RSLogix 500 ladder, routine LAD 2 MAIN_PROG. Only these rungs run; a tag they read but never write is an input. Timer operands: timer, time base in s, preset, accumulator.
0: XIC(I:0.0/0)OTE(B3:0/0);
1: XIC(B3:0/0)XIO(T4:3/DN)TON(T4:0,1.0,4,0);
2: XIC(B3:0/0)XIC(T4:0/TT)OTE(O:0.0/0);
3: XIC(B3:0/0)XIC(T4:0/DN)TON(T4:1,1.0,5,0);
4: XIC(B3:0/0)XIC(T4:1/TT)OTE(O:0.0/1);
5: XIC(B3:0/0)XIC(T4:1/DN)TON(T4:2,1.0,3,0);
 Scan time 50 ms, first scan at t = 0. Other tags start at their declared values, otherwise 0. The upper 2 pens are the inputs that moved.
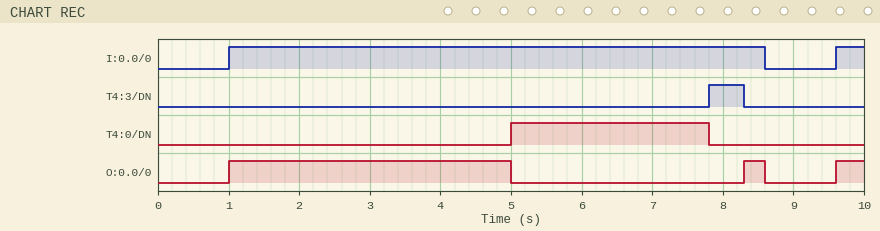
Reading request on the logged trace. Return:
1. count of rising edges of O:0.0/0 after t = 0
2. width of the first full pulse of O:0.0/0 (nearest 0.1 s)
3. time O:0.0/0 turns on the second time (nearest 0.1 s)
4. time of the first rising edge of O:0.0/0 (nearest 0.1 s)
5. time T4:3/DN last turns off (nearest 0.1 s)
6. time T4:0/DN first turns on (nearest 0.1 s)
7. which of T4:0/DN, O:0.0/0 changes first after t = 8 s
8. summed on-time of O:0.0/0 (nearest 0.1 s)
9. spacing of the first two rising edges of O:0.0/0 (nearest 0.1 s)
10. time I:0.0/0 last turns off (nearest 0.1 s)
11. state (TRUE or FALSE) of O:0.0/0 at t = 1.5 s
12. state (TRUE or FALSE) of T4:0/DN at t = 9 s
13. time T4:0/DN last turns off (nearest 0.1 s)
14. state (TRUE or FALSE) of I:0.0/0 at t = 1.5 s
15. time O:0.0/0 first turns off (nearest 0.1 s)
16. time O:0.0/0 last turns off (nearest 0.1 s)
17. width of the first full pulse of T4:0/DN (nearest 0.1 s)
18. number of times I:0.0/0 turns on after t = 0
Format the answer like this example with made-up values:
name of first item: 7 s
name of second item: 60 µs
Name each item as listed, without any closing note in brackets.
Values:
count of rising edges of O:0.0/0 after t = 0: 3
width of the first full pulse of O:0.0/0: 4.0 s
time O:0.0/0 turns on the second time: 8.3 s
time of the first rising edge of O:0.0/0: 1.0 s
time T4:3/DN last turns off: 8.3 s
time T4:0/DN first turns on: 5.0 s
which of T4:0/DN, O:0.0/0 changes first after t = 8 s: O:0.0/0
summed on-time of O:0.0/0: 4.7 s
spacing of the first two rising edges of O:0.0/0: 7.3 s
time I:0.0/0 last turns off: 8.6 s
state (TRUE or FALSE) of O:0.0/0 at t = 1.5 s: TRUE
state (TRUE or FALSE) of T4:0/DN at t = 9 s: FALSE
time T4:0/DN last turns off: 7.8 s
state (TRUE or FALSE) of I:0.0/0 at t = 1.5 s: TRUE
time O:0.0/0 first turns off: 5.0 s
time O:0.0/0 last turns off: 8.6 s
width of the first full pulse of T4:0/DN: 2.8 s
number of times I:0.0/0 turns on after t = 0: 2
